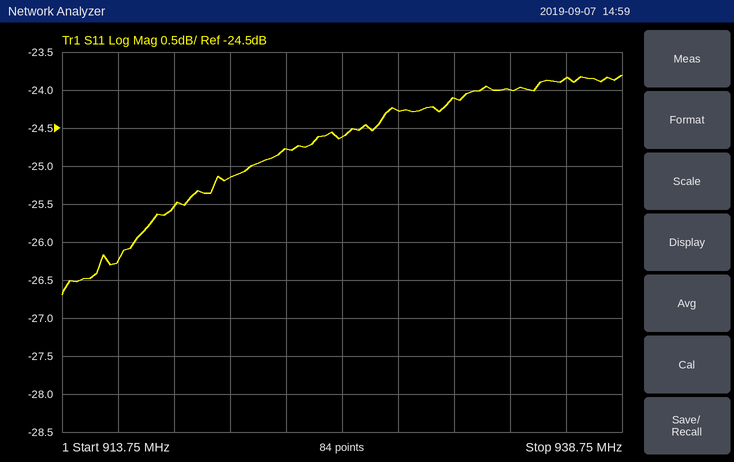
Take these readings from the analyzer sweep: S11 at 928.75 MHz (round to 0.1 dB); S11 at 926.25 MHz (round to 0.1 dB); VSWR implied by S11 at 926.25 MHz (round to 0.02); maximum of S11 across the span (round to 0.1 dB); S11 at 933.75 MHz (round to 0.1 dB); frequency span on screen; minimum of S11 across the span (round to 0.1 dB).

-24.3 dB
-24.6 dB
1.12
-23.8 dB
-24.0 dB
25 MHz
-26.7 dB
